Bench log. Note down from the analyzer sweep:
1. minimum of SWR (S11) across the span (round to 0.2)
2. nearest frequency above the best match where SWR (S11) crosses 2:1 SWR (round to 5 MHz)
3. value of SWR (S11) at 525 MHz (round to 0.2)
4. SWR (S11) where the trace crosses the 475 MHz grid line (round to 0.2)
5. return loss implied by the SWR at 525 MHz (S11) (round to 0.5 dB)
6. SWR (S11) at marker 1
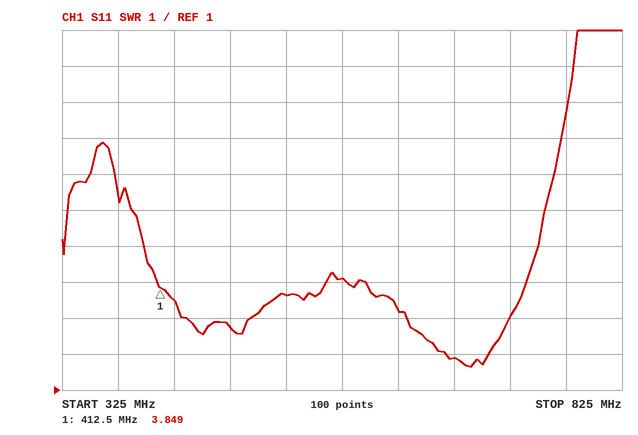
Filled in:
1.6
705 MHz
3.6
2.8
5.0 dB
3.849
